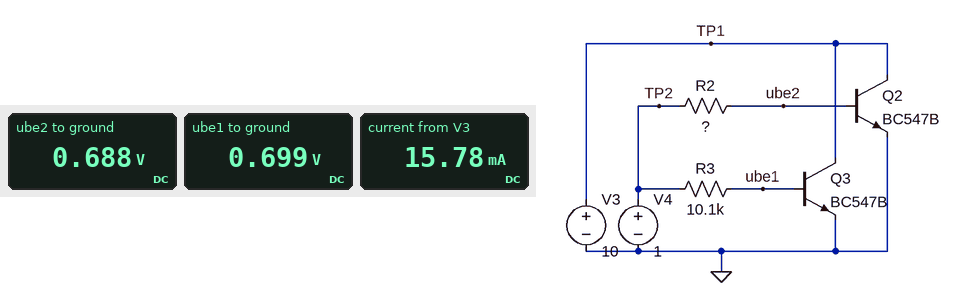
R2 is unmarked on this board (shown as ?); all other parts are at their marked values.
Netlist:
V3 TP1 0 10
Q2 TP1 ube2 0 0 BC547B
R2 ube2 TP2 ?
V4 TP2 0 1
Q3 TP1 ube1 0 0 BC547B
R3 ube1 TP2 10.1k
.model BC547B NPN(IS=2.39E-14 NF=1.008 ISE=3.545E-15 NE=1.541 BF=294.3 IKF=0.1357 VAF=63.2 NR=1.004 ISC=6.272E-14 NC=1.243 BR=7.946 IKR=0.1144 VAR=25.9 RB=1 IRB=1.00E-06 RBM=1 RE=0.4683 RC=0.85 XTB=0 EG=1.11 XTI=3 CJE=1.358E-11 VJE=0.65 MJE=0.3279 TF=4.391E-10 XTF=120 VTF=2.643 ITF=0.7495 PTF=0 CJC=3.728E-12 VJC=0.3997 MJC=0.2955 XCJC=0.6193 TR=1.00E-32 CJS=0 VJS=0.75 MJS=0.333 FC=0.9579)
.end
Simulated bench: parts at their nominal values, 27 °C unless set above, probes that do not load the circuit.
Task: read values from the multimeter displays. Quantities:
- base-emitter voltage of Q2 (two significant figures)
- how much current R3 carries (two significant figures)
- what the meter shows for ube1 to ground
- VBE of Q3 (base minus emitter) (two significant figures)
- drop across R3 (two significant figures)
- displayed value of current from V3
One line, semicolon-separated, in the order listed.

690 mV; 30 µA; 0.699 V; 700 mV; 300 mV; 15.78 mA
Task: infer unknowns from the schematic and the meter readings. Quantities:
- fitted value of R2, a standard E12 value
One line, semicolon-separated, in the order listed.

15 kΩ
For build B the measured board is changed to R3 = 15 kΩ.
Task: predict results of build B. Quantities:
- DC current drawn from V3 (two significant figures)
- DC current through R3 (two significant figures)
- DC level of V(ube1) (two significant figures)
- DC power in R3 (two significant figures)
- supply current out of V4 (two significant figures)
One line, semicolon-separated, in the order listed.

13 mA; 21 µA; 690 mV; 6.5 µW; 42 µA
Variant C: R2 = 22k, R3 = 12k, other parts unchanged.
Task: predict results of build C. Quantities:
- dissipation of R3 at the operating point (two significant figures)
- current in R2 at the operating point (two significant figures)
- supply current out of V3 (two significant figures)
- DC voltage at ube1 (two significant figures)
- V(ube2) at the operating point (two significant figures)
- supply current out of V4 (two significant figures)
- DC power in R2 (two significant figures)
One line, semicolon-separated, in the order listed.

7.8 µW; 15 µA; 13 mA; 690 mV; 680 mV; 40 µA; 4.7 µW
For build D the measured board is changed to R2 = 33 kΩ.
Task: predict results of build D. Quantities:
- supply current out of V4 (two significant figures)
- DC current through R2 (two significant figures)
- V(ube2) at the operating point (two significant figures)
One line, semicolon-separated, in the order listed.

40 µA; 10 µA; 670 mV
